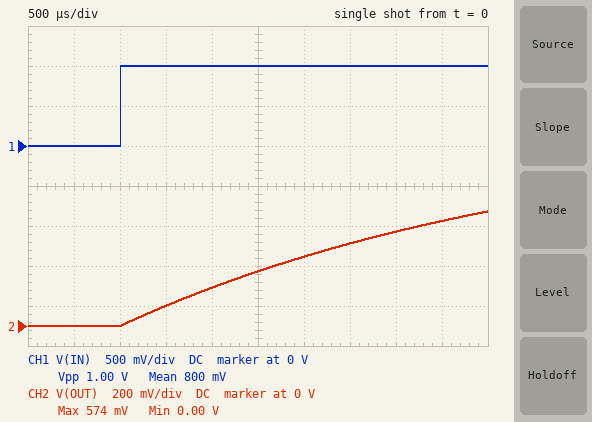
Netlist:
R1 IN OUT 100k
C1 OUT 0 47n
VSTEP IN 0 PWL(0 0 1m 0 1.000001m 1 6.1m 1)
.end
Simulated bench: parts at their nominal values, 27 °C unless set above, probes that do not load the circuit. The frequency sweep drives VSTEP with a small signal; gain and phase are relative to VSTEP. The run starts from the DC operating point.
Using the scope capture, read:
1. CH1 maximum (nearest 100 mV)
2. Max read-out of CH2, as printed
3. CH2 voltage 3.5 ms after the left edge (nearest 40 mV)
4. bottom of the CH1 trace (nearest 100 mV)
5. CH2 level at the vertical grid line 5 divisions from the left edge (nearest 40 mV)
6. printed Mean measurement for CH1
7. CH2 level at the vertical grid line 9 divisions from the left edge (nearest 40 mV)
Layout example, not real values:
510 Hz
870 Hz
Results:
1.0 V
574 mV
400 mV
0 V
280 mV
800 mV
520 mV
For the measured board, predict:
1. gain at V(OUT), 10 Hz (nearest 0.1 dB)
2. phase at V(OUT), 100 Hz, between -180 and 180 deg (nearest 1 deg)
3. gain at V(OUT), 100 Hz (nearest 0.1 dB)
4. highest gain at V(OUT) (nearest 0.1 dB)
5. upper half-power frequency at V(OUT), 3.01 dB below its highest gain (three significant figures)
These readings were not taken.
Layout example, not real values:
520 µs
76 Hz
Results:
-0.4 dB
-71 deg
-9.9 dB
0 dB
33.9 Hz
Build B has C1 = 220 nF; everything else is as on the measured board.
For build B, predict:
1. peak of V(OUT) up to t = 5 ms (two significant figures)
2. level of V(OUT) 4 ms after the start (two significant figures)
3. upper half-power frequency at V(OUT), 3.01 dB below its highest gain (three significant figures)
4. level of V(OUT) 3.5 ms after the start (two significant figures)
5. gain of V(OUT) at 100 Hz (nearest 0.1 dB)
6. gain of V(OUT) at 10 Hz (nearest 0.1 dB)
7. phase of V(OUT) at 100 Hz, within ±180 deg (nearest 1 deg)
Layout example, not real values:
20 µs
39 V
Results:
170 mV
130 mV
7.23 Hz
110 mV
-22.8 dB
-4.6 dB
-86 deg
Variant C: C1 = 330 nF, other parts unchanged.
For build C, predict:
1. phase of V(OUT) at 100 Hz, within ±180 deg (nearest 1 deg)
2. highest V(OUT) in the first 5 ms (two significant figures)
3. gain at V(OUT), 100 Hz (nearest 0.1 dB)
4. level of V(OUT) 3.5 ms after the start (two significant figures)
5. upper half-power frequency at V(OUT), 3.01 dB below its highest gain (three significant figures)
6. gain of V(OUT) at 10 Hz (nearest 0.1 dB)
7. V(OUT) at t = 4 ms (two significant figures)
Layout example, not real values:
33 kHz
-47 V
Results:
-87 deg
110 mV
-26.3 dB
73 mV
4.82 Hz
-7.2 dB
87 mV
